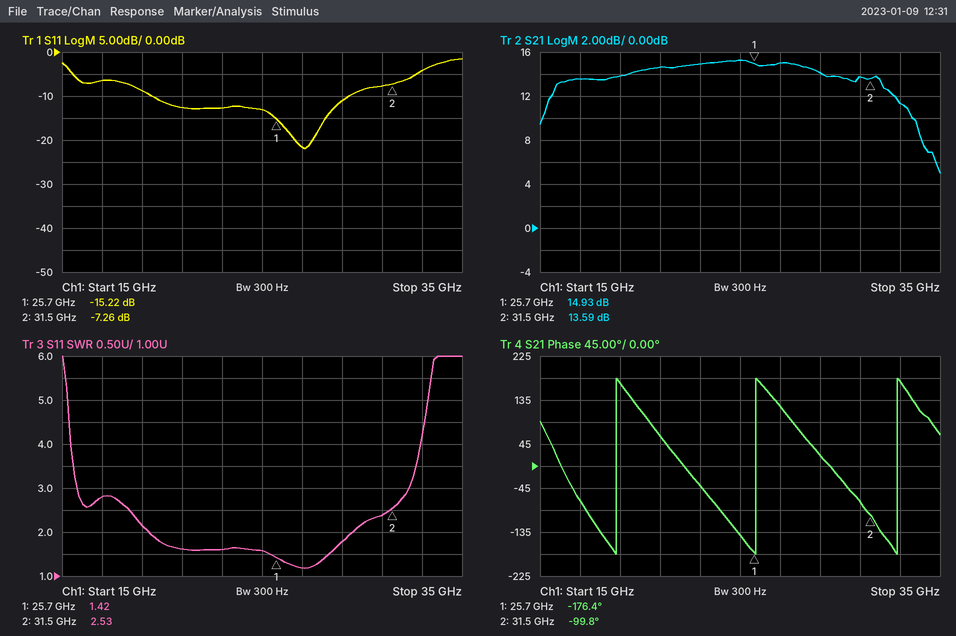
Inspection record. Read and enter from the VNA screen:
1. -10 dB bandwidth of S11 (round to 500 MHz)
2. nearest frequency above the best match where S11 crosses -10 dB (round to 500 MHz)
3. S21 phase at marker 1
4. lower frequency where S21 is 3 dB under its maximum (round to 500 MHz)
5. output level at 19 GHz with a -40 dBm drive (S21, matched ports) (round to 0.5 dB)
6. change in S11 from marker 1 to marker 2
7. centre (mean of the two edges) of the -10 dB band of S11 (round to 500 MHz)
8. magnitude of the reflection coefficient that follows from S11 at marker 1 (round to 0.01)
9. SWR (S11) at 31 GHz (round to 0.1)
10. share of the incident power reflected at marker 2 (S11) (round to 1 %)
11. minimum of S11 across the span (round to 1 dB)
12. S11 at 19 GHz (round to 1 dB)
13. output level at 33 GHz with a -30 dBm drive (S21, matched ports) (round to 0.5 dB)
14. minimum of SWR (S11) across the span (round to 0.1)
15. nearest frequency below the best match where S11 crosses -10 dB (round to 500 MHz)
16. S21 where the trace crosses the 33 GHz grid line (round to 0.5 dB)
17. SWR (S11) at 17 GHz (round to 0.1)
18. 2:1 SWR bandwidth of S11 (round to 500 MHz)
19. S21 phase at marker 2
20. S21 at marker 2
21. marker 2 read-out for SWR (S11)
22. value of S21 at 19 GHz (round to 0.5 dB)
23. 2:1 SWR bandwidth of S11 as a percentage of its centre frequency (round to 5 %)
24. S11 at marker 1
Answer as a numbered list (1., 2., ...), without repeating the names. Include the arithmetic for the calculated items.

1. 29.5 GHz − 19.5 GHz = 10.0 GHz
2. 29.5 GHz
3. -176.4°
4. 15.5 GHz
5. -40 dBm + (14.0 dB) = -26.0 dBm
6. -7.26 − (-15.22) = 7.96 dB
7. 24.5 GHz
8. 10^(-15.22/20) ≈ 0.17
9. 2.4
10. 10^(-7.26/10) ≈ 19 %
11. -22 dB
12. -9 dB
13. -30 dBm + (11.5 dB) = -18.5 dBm
14. 1.2
15. 19.5 GHz
16. 11.5 dB
17. 2.8
18. 29.5 GHz − 19.5 GHz = 10.0 GHz
19. -99.8°
20. 13.59 dB
21. 2.53
22. 14.0 dB
23. 10 GHz / 24.5 GHz ≈ 40.8 %, so 40 % to the nearest 5 %
24. -15.22 dB
